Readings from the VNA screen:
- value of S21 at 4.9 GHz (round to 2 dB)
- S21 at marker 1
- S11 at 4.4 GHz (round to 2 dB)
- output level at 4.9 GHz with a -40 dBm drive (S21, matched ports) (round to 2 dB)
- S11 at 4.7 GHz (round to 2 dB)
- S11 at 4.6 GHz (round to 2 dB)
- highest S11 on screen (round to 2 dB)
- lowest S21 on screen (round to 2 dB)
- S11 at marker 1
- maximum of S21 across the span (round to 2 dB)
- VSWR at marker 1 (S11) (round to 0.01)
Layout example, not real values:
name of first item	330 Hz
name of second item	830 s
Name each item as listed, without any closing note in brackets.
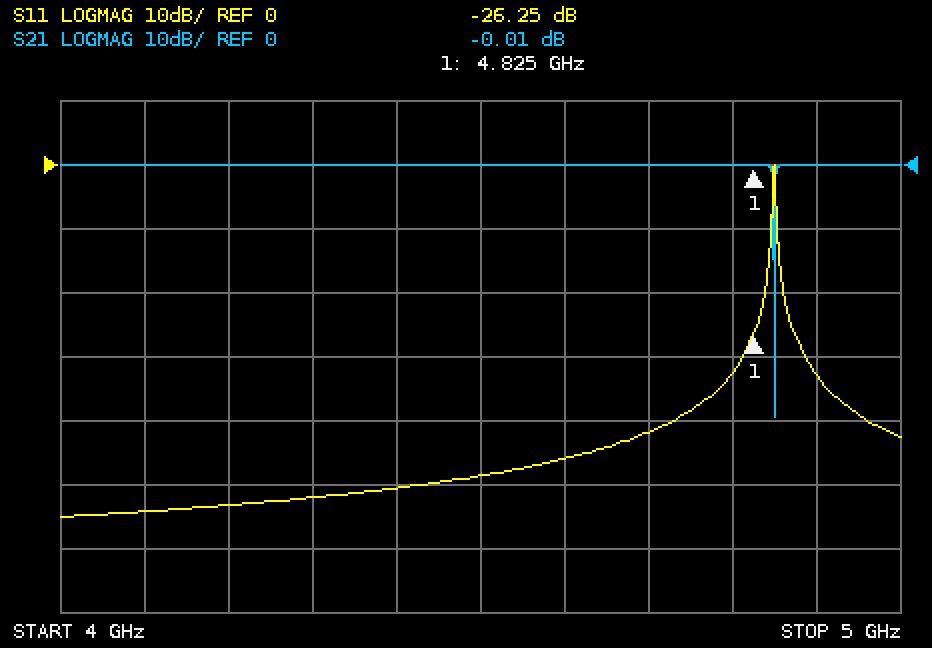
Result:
value of S21 at 4.9 GHz	0 dB
S21 at marker 1	-0.01 dB
S11 at 4.4 GHz	-50 dB
output level at 4.9 GHz with a -40 dBm drive (S21, matched ports)	-40 dBm
S11 at 4.7 GHz	-42 dB
S11 at 4.6 GHz	-46 dB
highest S11 on screen	0 dB
lowest S21 on screen	-40 dB
S11 at marker 1	-26.25 dB
maximum of S21 across the span	0 dB
VSWR at marker 1 (S11)	1.10
